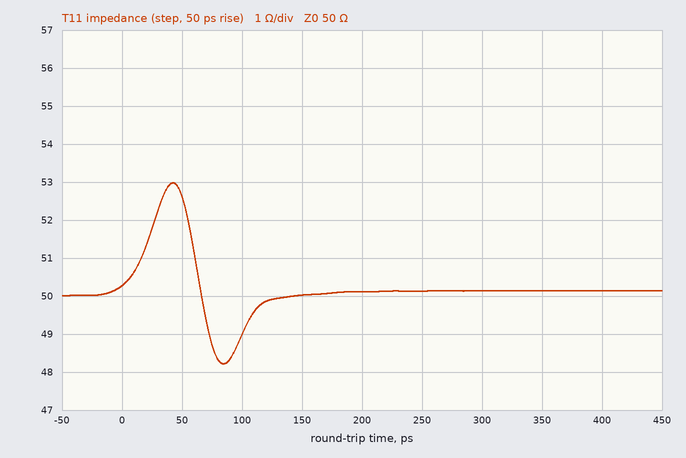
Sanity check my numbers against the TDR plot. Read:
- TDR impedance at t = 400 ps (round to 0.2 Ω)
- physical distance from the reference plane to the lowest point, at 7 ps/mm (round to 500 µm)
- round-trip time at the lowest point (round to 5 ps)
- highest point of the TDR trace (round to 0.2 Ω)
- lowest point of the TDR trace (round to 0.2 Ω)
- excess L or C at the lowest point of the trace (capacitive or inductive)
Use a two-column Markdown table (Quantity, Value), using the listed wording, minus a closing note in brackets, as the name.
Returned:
| Quantity | Value |
|---|---|
| TDR impedance at t = 400 ps | 50.2 Ω |
| physical distance from the reference plane to the lowest point, at 7 ps/mm | 6.0 mm |
| round-trip time at the lowest point | 85 ps |
| highest point of the TDR trace | 53.0 Ω |
| lowest point of the TDR trace | 48.2 Ω |
| excess L or C at the lowest point of the trace | capacitive |
